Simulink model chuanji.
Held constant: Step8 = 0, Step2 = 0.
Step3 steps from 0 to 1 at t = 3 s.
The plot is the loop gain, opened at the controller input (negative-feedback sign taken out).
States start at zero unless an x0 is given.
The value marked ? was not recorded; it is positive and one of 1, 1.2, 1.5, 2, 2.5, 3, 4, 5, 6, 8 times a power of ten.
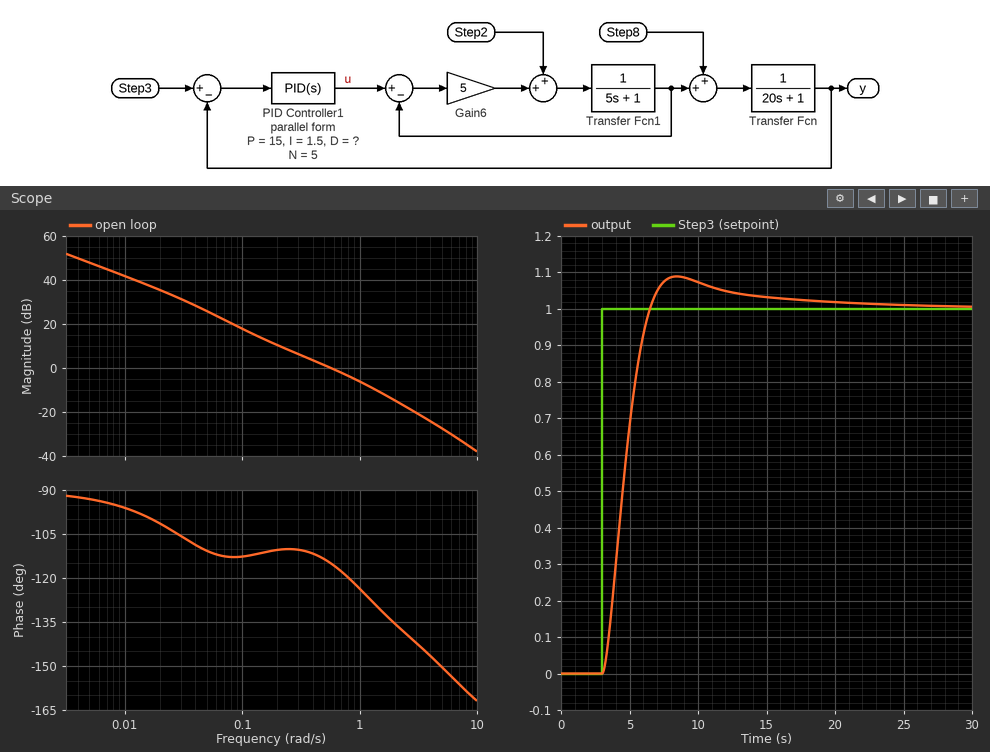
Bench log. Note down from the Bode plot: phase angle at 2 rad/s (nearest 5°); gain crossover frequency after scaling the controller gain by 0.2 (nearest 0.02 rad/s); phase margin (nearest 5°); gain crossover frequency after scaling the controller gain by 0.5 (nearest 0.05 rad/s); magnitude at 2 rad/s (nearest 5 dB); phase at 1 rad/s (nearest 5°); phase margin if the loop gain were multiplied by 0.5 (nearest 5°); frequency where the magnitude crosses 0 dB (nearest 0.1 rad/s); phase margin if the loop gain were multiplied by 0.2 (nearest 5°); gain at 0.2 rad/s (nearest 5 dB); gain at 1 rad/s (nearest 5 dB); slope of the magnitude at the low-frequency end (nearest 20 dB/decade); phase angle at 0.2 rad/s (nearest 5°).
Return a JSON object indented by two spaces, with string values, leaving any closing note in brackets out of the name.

{
  "phase angle at 2 rad/s": "-135°",
  "gain crossover frequency after scaling the controller gain by 0.2": "0.14 rad/s",
  "phase margin": "65°",
  "gain crossover frequency after scaling the controller gain by 0.5": "0.30 rad/s",
  "magnitude at 2 rad/s": "-15 dB",
  "phase at 1 rad/s": "-125°",
  "phase margin if the loop gain were multiplied by 0.5": "70°",
  "frequency where the magnitude crosses 0 dB": "0.6 rad/s",
  "phase margin if the loop gain were multiplied by 0.2": "70°",
  "gain at 0.2 rad/s": "10 dB",
  "gain at 1 rad/s": "-5 dB",
  "slope of the magnitude at the low-frequency end": "-20 dB/decade",
  "phase angle at 0.2 rad/s": "-110°"
}
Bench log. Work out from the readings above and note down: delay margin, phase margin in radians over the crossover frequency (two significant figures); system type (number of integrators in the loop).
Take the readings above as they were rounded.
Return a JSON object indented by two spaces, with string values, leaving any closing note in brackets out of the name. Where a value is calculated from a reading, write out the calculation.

{
  "delay margin, phase margin in radians over the crossover frequency": "65 × π / 180 / 0.6 = 1.9 s",
  "system type": "1"
}
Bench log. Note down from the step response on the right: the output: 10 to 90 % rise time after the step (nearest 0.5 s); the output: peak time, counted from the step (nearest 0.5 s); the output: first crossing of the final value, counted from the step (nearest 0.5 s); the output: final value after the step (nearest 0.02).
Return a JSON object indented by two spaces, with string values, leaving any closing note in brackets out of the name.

{
  "the output: 10 to 90 % rise time after the step": "2.5 s",
  "the output: peak time, counted from the step": "5.5 s",
  "the output: first crossing of the final value, counted from the step": "3.5 s",
  "the output: final value after the step": "1.00"
}
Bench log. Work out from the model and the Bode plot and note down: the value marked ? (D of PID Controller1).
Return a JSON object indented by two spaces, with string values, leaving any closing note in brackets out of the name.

{
  "the value marked ?": "2.5"
}
